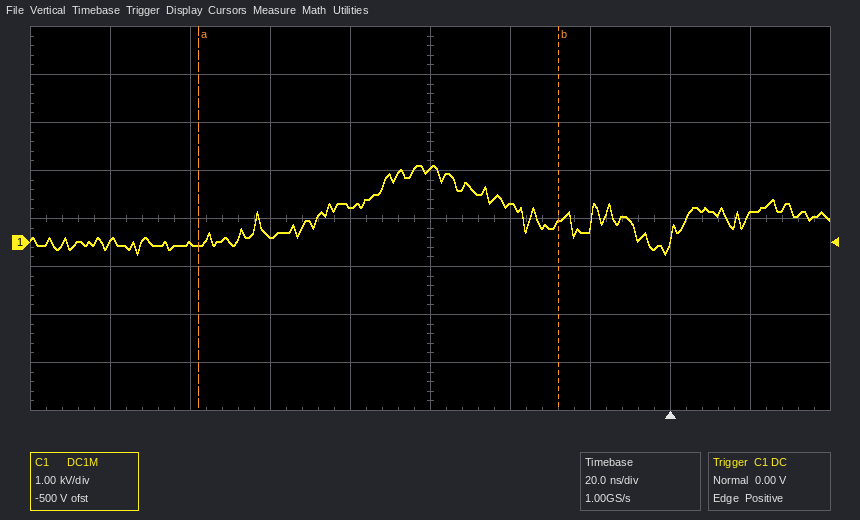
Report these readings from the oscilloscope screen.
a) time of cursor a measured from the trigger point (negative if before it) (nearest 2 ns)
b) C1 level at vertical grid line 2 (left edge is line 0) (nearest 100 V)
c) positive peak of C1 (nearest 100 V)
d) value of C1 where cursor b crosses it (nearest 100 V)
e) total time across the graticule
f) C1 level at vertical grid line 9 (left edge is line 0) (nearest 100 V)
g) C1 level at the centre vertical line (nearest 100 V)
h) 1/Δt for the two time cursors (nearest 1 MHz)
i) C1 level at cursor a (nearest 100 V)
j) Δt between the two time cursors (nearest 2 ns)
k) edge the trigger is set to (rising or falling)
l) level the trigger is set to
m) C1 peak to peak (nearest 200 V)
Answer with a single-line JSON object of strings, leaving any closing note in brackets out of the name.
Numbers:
{"time of cursor a measured from the trigger point (negative if before it)": "-118 ns", "C1 level at vertical grid line 2 (left edge is line 0)": "0.0 kV", "positive peak of C1": "1.6 kV", "value of C1 where cursor b crosses it": "400 V", "total time across the graticule": "200 ns", "C1 level at vertical grid line 9 (left edge is line 0)": "600 V", "C1 level at the centre vertical line": "1.5 kV", "1/Δt for the two time cursors": "11 MHz", "C1 level at cursor a": "-100 V", "Δt between the two time cursors": "90 ns", "edge the trigger is set to": "rising", "level the trigger is set to": "0.00 V", "C1 peak to peak": "1.8 kV"}
